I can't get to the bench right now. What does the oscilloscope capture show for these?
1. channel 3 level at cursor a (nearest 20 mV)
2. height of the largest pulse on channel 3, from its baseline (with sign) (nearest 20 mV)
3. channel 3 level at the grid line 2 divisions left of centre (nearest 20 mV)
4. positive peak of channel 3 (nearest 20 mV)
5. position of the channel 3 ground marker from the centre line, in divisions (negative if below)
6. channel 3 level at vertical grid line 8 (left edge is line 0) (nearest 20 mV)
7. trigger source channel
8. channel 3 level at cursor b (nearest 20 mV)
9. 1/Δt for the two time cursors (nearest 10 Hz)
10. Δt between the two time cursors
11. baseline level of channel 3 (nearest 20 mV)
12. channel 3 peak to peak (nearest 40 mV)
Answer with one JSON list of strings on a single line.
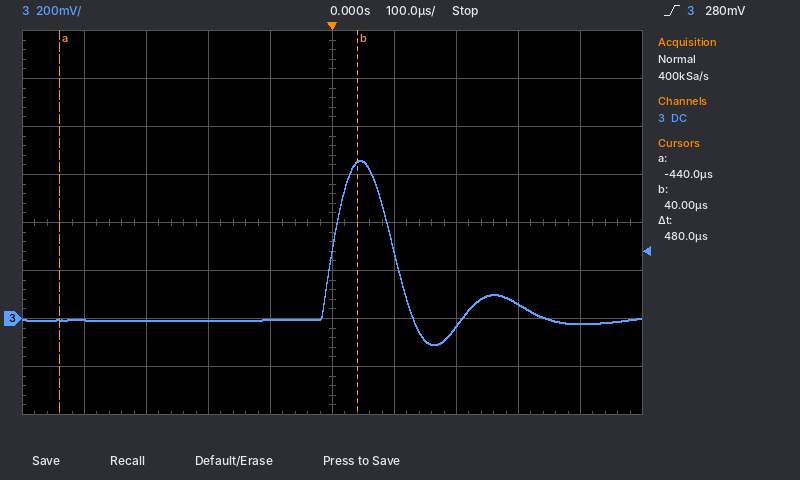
["0 mV", "+660 mV", "0 mV", "660 mV", "-2.0 div", "60 mV", "channel 3", "640 mV", "2.08 kHz", "480 µs", "0 mV", "760 mV"]
